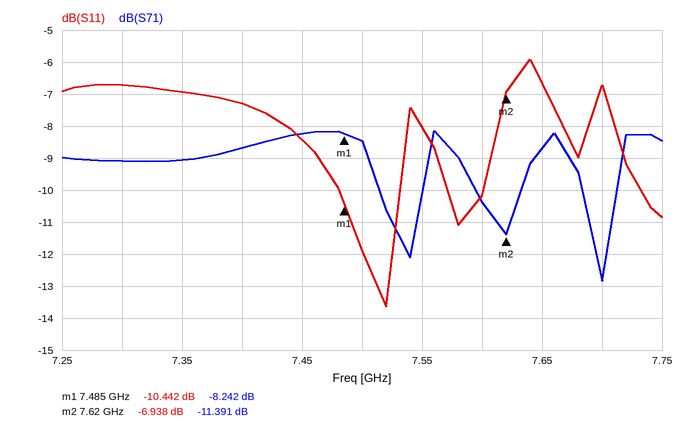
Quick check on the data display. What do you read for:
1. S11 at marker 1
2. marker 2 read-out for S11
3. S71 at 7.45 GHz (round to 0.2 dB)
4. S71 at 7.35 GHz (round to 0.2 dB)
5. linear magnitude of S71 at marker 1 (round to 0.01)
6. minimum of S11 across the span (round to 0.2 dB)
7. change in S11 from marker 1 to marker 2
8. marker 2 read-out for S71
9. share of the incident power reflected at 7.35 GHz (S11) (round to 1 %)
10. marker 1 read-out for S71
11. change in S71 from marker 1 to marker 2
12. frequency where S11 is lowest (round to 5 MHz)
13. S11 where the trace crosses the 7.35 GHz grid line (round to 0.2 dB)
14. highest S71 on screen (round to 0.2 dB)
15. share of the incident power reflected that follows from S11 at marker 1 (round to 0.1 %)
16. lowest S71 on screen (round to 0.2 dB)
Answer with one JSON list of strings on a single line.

["-10.442 dB", "-6.938 dB", "-8.2 dB", "-9.0 dB", "0.39", "-13.6 dB", "3.504 dB", "-11.391 dB", "20 %", "-8.242 dB", "-3.149 dB", "7.520 GHz", "-7.0 dB", "-8.2 dB", "9.0 %", "-12.8 dB"]
